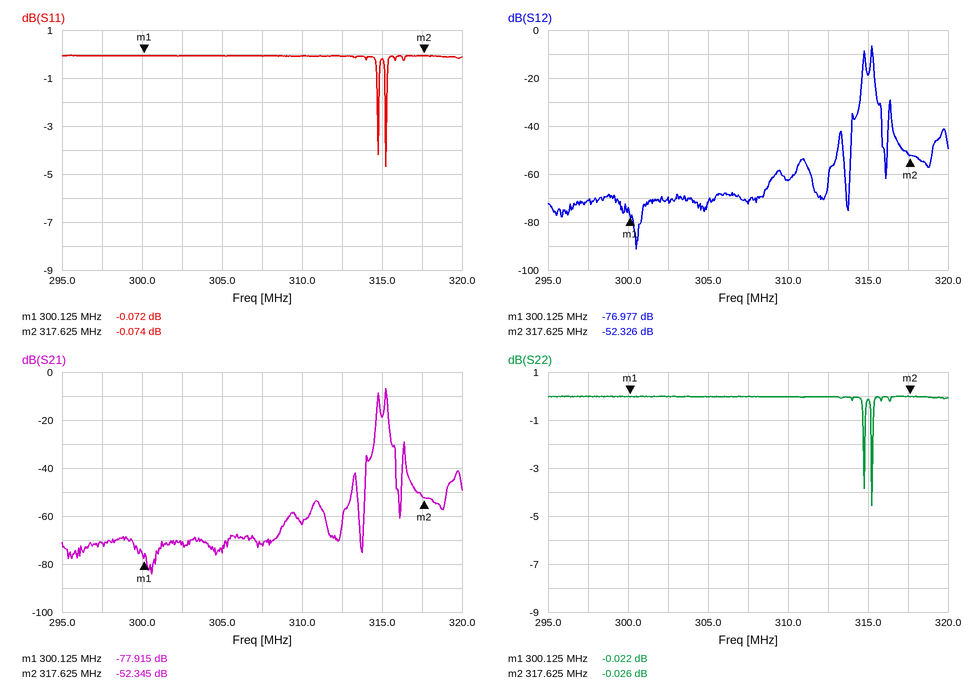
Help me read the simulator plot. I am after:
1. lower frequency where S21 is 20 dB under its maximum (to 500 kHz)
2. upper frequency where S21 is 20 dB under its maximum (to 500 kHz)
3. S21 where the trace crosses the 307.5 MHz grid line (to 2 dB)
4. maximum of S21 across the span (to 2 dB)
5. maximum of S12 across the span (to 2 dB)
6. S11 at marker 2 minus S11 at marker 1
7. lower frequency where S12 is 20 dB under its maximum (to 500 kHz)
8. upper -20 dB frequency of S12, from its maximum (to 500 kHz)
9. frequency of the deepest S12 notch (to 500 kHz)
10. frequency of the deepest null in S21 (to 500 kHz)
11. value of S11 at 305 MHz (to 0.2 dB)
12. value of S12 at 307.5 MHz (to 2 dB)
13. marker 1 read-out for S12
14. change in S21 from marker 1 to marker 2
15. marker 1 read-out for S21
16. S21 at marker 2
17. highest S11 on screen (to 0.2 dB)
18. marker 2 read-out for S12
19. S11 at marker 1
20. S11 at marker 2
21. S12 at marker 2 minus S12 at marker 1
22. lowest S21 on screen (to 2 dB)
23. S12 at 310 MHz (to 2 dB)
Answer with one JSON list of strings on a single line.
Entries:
["314.5 MHz", "315.5 MHz", "-72 dB", "-6 dB", "-6 dB", "-0.002 dB", "314.5 MHz", "315.5 MHz", "300.5 MHz", "300.5 MHz", "0.0 dB", "-72 dB", "-76.977 dB", "25.570 dB", "-77.915 dB", "-52.345 dB", "0.0 dB", "-52.326 dB", "-0.072 dB", "-0.074 dB", "24.651 dB", "-84 dB", "-62 dB"]
